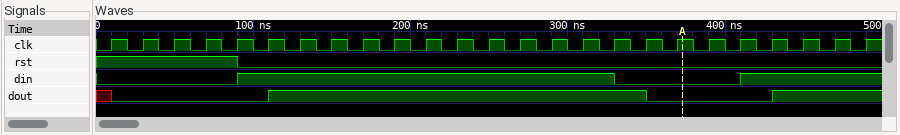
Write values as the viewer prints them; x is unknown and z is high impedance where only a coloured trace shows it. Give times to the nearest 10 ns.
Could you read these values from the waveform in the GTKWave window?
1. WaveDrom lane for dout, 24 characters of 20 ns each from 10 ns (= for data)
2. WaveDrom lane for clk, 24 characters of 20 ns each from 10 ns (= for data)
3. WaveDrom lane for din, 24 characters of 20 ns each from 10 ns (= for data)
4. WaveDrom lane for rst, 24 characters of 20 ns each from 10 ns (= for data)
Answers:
{name: 'dout', wave: '0....1...........0...1..'}
{name: 'clk', wave: 'p.......................'}
{name: 'din', wave: '0...1...........0...1...'}
{name: 'rst', wave: '1...0...................'}
